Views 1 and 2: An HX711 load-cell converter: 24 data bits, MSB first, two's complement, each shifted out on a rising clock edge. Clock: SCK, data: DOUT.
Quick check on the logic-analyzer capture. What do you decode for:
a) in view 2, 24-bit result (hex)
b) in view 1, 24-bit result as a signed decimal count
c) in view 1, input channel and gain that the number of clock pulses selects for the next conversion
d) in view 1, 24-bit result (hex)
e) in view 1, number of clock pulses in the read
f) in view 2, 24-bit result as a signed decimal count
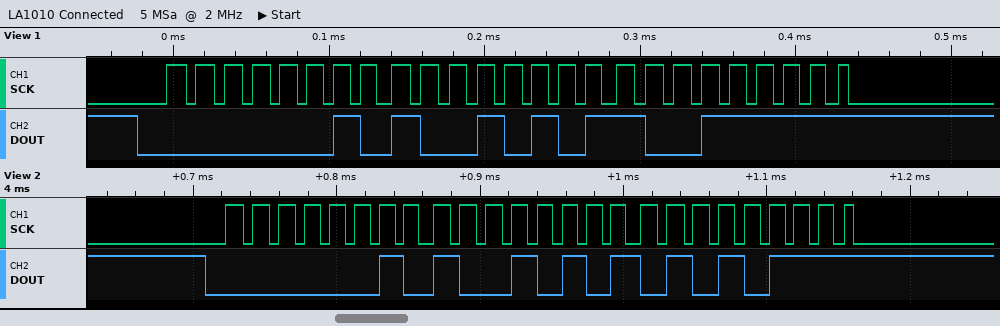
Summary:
0x029557
169375
channel A, gain 128
0x02959F
25
169303
